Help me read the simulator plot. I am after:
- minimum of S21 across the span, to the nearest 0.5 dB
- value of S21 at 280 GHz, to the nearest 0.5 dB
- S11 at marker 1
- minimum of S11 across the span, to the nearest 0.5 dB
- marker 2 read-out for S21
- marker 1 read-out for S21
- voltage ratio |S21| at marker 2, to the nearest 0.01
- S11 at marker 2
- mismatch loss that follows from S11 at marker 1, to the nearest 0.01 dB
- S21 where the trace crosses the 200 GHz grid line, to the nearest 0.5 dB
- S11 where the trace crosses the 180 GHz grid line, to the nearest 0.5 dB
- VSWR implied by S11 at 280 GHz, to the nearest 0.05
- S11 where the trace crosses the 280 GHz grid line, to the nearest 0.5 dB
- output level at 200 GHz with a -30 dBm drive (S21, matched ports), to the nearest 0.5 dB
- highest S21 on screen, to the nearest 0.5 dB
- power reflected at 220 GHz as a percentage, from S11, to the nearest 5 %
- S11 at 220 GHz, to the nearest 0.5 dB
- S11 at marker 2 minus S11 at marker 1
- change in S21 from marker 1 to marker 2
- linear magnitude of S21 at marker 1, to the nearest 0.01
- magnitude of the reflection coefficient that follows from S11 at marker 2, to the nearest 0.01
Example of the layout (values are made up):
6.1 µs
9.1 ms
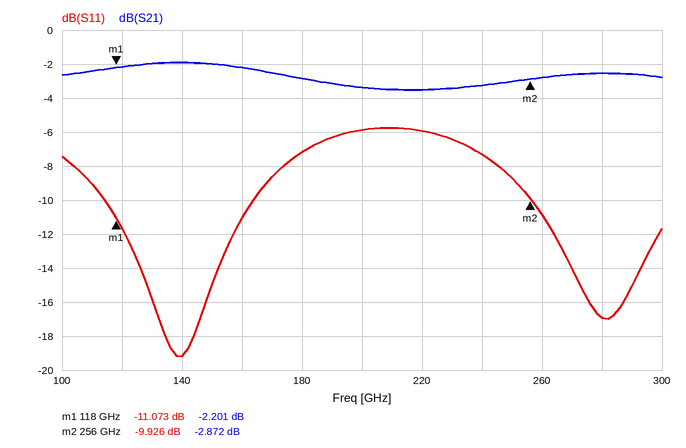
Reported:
-3.5 dB
-2.5 dB
-11.073 dB
-19.0 dB
-2.872 dB
-2.201 dB
0.72
-9.926 dB
0.35 dB
-3.5 dB
-7.0 dB
1.35
-17.0 dB
-33.5 dBm
-2.0 dB
25 %
-6.0 dB
1.147 dB
-0.671 dB
0.78
0.32
